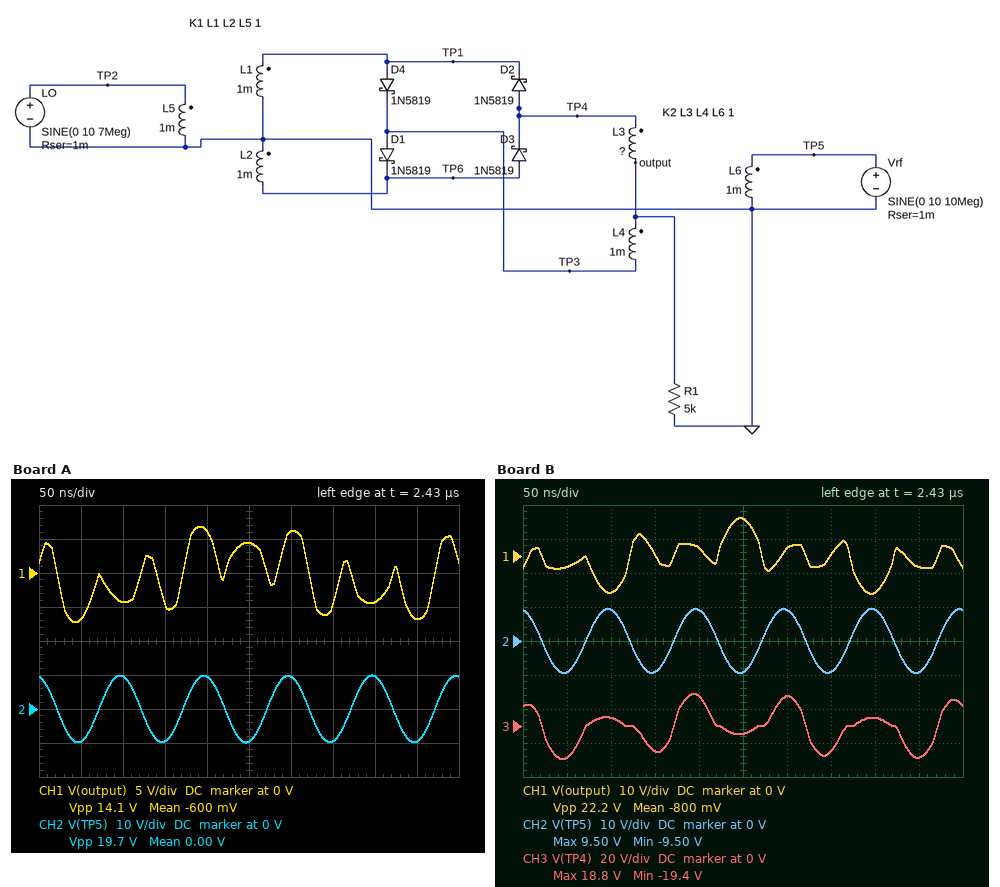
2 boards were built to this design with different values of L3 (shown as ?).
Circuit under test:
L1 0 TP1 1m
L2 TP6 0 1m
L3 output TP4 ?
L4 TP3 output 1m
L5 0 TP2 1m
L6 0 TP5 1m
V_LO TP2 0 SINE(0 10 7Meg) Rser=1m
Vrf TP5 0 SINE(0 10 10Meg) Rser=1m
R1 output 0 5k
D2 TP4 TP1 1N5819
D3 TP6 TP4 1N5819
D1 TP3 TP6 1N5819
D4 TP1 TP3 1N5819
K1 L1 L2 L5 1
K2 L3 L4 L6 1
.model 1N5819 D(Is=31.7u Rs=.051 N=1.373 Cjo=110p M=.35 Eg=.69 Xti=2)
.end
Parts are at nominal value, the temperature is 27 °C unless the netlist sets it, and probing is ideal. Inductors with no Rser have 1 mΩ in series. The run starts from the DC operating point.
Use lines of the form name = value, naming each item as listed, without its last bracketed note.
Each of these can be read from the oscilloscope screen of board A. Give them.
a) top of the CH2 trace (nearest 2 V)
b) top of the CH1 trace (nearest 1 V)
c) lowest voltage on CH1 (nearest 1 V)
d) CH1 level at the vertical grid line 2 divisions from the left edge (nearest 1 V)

top of the CH2 trace = 10 V
top of the CH1 trace = 7 V
lowest voltage on CH1 = -7 V
CH1 level at the vertical grid line 2 divisions from the left edge = -4 V
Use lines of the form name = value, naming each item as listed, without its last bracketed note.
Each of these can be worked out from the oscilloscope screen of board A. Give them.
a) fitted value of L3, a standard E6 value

fitted value of L3, a standard E6 value = 470 µH
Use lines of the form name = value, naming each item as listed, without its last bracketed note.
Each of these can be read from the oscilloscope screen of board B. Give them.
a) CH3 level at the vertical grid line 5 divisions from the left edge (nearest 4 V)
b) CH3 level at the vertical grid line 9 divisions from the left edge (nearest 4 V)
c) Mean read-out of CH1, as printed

CH3 level at the vertical grid line 5 divisions from the left edge = -4 V
CH3 level at the vertical grid line 9 divisions from the left edge = -20 V
Mean read-out of CH1, as printed = -800 mV
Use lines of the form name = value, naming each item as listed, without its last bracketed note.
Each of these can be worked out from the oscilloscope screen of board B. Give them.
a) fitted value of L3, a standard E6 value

fitted value of L3, a standard E6 value = 3.3 mH
